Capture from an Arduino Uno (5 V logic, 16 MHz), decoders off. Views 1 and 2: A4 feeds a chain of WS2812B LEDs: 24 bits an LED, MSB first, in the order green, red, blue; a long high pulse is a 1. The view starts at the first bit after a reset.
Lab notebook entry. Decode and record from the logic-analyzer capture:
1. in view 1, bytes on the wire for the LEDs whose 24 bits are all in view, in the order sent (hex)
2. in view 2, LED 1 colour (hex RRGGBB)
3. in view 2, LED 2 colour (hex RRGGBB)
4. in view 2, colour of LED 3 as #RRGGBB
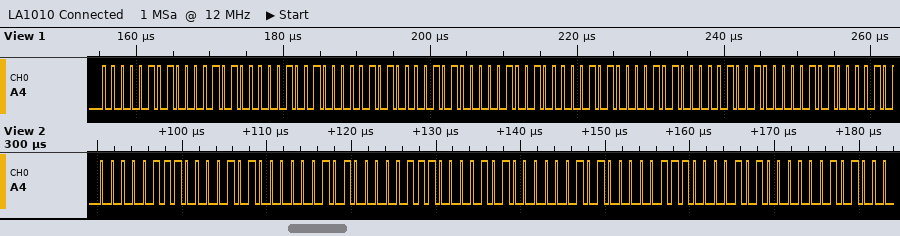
05 0A 09 05 0A 09 05 0A 09
#0A0705
#0A0705
#0A0705
